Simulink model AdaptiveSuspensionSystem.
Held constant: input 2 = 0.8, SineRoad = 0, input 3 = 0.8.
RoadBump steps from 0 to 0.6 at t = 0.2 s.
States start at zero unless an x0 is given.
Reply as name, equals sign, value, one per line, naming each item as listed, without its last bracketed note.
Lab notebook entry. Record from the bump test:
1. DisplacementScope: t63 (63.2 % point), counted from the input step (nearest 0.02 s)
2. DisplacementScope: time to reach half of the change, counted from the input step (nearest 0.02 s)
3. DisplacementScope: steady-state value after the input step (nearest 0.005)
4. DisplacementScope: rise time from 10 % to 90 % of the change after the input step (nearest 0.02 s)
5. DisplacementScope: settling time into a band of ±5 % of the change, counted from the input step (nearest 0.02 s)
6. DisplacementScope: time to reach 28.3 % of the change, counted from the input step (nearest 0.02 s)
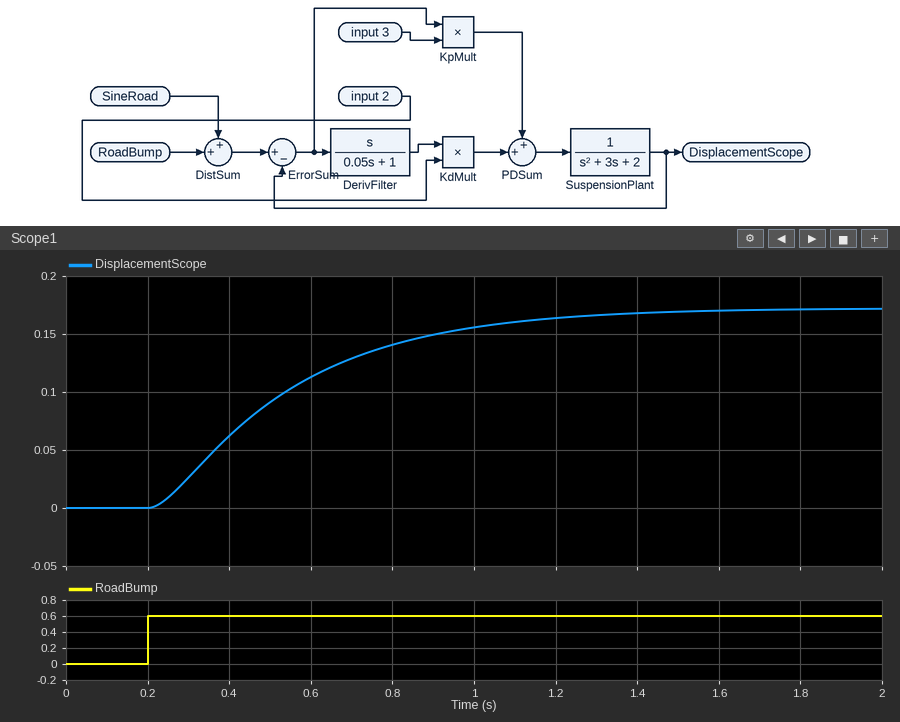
DisplacementScope: t63 (63.2 % point), counted from the input step = 0.38 s
DisplacementScope: time to reach half of the change, counted from the input step = 0.28 s
DisplacementScope: steady-state value after the input step = 0.170
DisplacementScope: rise time from 10 % to 90 % of the change after the input step = 0.70 s
DisplacementScope: settling time into a band of ±5 % of the change, counted from the input step = 0.98 s
DisplacementScope: time to reach 28.3 % of the change, counted from the input step = 0.16 s
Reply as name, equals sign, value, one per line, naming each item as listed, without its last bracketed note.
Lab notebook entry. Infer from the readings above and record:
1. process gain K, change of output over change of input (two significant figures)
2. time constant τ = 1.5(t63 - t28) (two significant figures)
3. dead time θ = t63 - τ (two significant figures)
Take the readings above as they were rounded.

process gain K, change of output over change of input = 0.28
time constant τ = 1.5(t63 - t28) = 0.33 s
dead time θ = t63 - τ = 0.050 s
